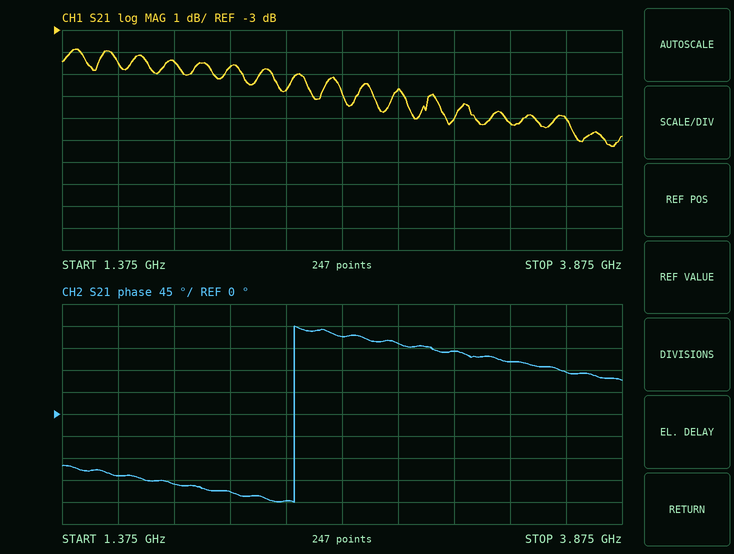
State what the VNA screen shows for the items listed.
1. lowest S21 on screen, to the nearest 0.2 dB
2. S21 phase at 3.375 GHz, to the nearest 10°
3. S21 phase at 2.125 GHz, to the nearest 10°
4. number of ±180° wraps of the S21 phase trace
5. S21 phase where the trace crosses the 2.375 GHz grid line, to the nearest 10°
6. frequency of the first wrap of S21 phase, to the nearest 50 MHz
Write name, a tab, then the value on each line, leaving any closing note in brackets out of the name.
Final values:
lowest S21 on screen, to the nearest 0.2 dB	-8.2 dB
S21 phase at 3.375 GHz, to the nearest 10°	110°
S21 phase at 2.125 GHz, to the nearest 10°	-160°
number of ±180° wraps of the S21 phase trace	1
S21 phase where the trace crosses the 2.375 GHz grid line, to the nearest 10°	-180°
frequency of the first wrap of S21 phase, to the nearest 50 MHz	2.40 GHz
